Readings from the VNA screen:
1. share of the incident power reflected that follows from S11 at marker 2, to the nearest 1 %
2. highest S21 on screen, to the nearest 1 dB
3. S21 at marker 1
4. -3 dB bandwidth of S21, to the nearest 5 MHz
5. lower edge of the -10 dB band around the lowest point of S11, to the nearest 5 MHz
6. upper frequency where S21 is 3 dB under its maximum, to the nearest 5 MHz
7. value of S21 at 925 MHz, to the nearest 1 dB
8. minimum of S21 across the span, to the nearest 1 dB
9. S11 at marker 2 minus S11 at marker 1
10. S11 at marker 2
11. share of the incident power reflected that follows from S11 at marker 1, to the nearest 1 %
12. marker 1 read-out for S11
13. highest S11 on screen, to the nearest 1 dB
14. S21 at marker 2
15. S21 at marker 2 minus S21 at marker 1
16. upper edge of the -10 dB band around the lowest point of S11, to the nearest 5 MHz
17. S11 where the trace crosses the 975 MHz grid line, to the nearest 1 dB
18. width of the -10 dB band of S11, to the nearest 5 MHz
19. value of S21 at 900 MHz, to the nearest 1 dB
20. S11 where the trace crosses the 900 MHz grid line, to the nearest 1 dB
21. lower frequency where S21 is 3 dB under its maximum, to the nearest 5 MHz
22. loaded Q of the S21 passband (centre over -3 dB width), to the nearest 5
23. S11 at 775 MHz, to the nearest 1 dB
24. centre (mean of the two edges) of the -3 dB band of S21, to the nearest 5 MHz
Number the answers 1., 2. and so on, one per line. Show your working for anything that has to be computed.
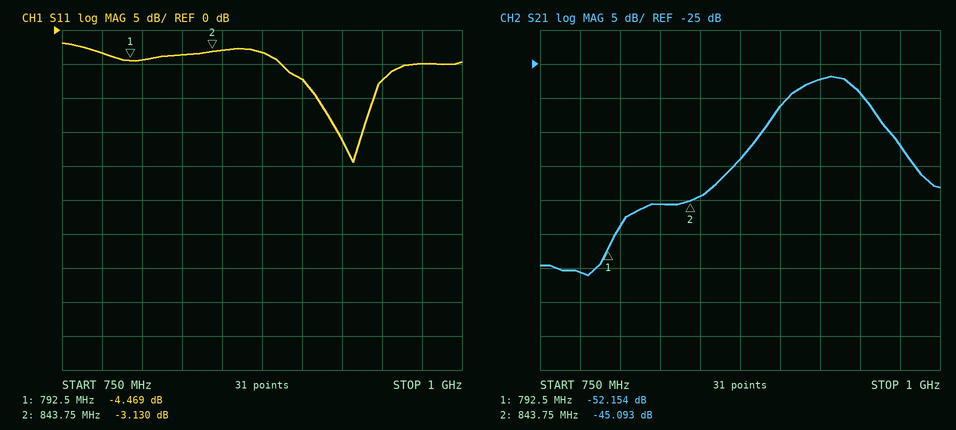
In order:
1. 10^(-3.13/10) ≈ 49 %
2. -27 dB
3. -52.154 dB
4. 950 MHz − 905 MHz = 45 MHz
5. 910 MHz
6. 950 MHz
7. -27 dB
8. -56 dB
9. -3.13 − (-4.469) = 1.339 dB
10. -3.130 dB
11. 10^(-4.469/10) ≈ 36 %
12. -4.469 dB
13. -2 dB
14. -45.093 dB
15. -45.093 − (-52.154) = 7.061 dB
16. 945 MHz
17. -5 dB
18. 945 MHz − 910 MHz = 35 MHz
19. -31 dB
20. -7 dB
21. 905 MHz
22. 927.5 MHz / 45 MHz ≈ 20.6, so 20 to the nearest 5
23. -3 dB
24. 930 MHz
